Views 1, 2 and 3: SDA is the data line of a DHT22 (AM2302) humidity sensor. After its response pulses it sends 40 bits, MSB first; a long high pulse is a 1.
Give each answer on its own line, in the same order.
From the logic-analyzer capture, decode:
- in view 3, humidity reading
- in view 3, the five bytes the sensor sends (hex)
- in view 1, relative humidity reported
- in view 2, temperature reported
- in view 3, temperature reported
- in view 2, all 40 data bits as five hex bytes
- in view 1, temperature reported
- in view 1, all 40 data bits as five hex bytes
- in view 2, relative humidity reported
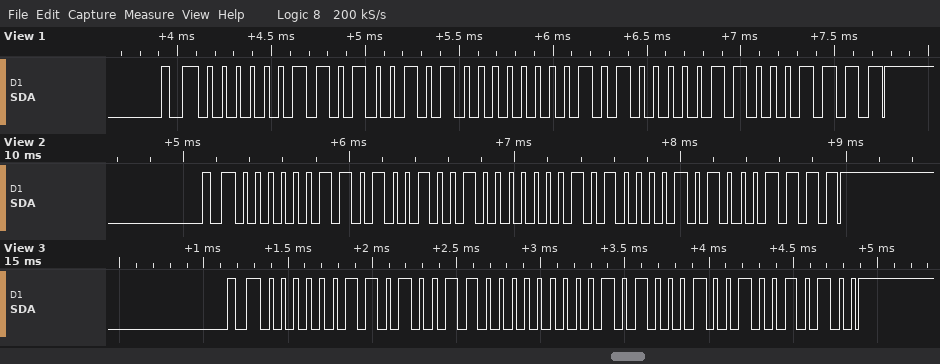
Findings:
84.4 %
03 4C 01 44 94
84.2 %
32.2 °C
32.4 °C
03 49 01 42 8F
32.1 °C
03 4A 01 41 8F
84.1 %
